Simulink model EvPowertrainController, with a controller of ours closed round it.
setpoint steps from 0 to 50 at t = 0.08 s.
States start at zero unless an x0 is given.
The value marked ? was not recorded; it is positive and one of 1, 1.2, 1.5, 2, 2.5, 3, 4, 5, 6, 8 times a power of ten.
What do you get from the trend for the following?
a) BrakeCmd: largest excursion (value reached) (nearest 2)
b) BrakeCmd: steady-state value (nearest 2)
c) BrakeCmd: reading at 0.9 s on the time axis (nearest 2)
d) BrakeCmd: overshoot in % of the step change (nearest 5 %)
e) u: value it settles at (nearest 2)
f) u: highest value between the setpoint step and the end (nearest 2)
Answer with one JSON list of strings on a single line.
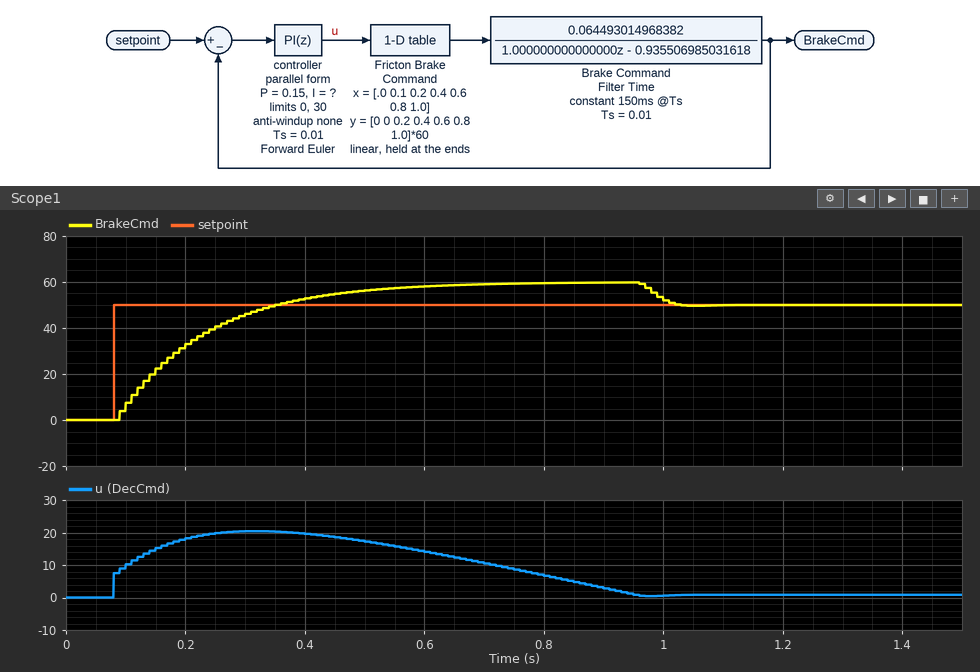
["60", "50", "60", "20 %", "0", "20"]
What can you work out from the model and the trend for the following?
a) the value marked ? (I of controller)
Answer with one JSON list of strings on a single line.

["4"]
